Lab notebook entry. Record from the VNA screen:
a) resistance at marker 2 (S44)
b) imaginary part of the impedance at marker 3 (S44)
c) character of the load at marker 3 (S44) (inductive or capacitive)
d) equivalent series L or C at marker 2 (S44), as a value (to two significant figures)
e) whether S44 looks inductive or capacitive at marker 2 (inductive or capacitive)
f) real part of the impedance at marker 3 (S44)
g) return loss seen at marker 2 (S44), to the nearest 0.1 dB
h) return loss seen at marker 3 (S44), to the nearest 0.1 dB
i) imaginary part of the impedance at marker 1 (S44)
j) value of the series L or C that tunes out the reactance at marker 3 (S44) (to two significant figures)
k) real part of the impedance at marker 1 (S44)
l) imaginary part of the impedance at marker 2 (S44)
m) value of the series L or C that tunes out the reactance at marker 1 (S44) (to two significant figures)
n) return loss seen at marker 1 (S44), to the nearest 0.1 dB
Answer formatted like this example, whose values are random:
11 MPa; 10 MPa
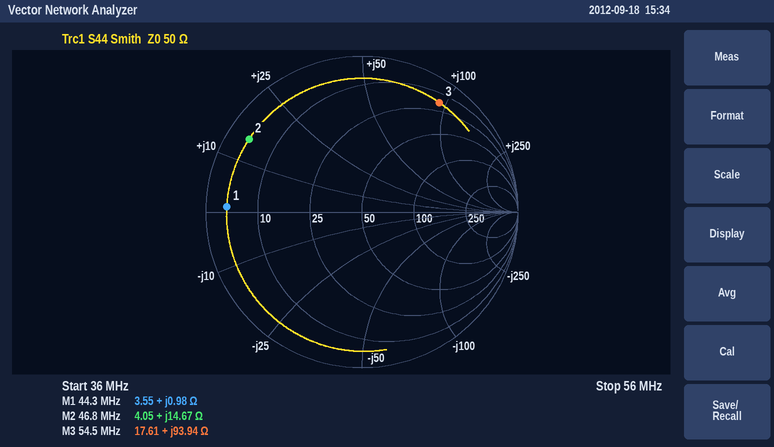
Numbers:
4.05 Ω; +93.94 Ω; inductive; 50 nH; inductive; 17.61 Ω; 1.3 dB; 1.3 dB; +0.98 Ω; 31 pF; 3.55 Ω; +14.67 Ω; 3.7 nF; 1.2 dB
